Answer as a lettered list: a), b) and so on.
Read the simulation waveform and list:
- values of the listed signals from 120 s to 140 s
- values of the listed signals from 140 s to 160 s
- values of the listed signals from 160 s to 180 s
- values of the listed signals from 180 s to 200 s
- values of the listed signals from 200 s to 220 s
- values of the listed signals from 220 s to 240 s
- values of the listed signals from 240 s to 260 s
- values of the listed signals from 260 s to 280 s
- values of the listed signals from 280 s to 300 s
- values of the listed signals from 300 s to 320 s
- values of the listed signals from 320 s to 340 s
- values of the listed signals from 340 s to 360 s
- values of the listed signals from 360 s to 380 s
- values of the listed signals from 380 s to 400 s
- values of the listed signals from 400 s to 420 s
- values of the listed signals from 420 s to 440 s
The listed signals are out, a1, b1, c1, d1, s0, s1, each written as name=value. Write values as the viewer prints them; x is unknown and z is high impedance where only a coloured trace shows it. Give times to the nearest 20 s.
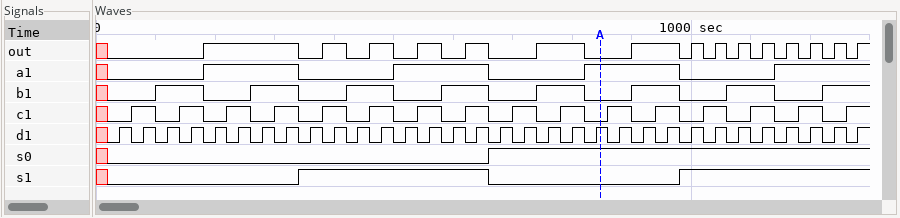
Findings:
a) out=0, a1=0, b1=1, c1=0, d1=1, s0=0, s1=0
b) out=0, a1=0, b1=1, c1=1, d1=0, s0=0, s1=0
c) out=0, a1=0, b1=1, c1=1, d1=1, s0=0, s1=0
d) out=1, a1=1, b1=0, c1=0, d1=0, s0=0, s1=0
e) out=1, a1=1, b1=0, c1=0, d1=1, s0=0, s1=0
f) out=1, a1=1, b1=0, c1=1, d1=0, s0=0, s1=0
g) out=1, a1=1, b1=0, c1=1, d1=1, s0=0, s1=0
h) out=1, a1=1, b1=1, c1=0, d1=0, s0=0, s1=0
i) out=1, a1=1, b1=1, c1=0, d1=1, s0=0, s1=0
j) out=1, a1=1, b1=1, c1=1, d1=0, s0=0, s1=0
k) out=1, a1=1, b1=1, c1=1, d1=1, s0=0, s1=0
l) out=0, a1=0, b1=0, c1=0, d1=0, s0=0, s1=1
m) out=0, a1=0, b1=0, c1=0, d1=1, s0=0, s1=1
n) out=1, a1=0, b1=0, c1=1, d1=0, s0=0, s1=1
o) out=1, a1=0, b1=0, c1=1, d1=1, s0=0, s1=1
p) out=0, a1=0, b1=1, c1=0, d1=0, s0=0, s1=1
